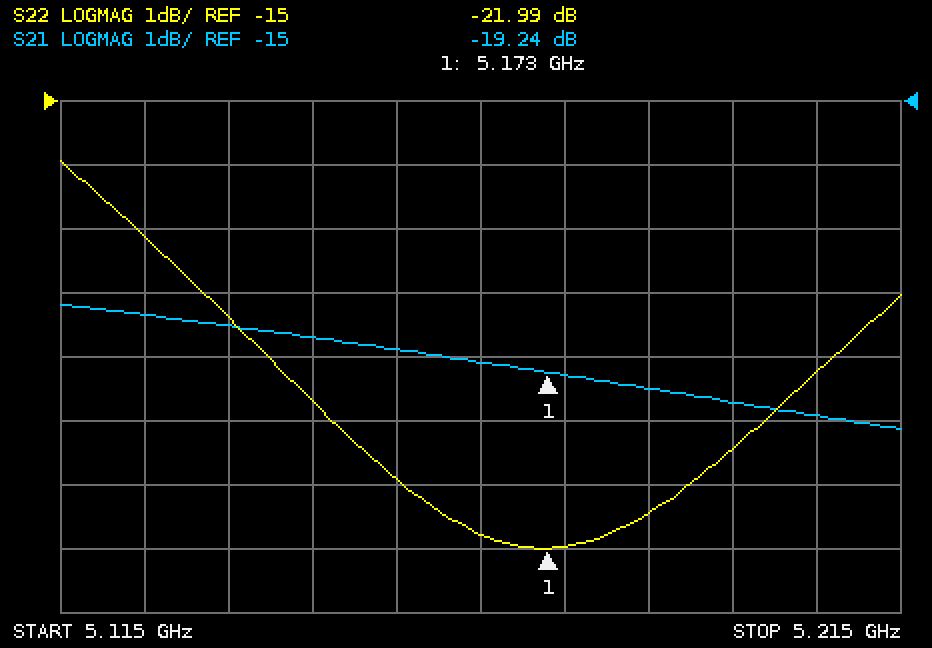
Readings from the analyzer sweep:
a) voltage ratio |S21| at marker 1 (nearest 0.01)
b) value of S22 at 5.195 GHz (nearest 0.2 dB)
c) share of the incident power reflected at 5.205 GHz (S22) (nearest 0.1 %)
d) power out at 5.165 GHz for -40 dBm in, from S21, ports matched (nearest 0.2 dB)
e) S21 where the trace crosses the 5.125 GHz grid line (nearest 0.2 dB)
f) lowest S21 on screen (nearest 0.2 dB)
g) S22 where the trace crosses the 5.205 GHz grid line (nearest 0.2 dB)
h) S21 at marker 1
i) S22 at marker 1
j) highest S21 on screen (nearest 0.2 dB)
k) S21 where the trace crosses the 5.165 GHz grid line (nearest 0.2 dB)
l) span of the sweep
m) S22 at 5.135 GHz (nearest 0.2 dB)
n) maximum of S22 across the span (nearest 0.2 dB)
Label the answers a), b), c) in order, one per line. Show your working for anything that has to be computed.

a) 10^(-19.24/20) ≈ 0.11
b) -20.4 dB
c) 10^(-19.2/10) ≈ 1.2 %
d) -40 dBm + (-19.0 dB) = -59.0 dBm
e) -18.4 dB
f) -20.2 dB
g) -19.2 dB
h) -19.24 dB
i) -21.99 dB
j) -18.2 dB
k) -19.0 dB
l) 100 MHz
m) -18.4 dB
n) -16.0 dB
